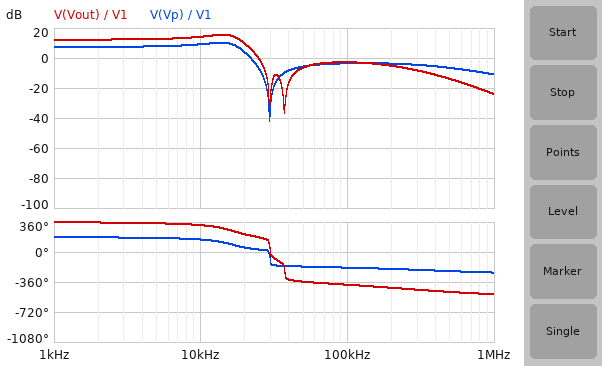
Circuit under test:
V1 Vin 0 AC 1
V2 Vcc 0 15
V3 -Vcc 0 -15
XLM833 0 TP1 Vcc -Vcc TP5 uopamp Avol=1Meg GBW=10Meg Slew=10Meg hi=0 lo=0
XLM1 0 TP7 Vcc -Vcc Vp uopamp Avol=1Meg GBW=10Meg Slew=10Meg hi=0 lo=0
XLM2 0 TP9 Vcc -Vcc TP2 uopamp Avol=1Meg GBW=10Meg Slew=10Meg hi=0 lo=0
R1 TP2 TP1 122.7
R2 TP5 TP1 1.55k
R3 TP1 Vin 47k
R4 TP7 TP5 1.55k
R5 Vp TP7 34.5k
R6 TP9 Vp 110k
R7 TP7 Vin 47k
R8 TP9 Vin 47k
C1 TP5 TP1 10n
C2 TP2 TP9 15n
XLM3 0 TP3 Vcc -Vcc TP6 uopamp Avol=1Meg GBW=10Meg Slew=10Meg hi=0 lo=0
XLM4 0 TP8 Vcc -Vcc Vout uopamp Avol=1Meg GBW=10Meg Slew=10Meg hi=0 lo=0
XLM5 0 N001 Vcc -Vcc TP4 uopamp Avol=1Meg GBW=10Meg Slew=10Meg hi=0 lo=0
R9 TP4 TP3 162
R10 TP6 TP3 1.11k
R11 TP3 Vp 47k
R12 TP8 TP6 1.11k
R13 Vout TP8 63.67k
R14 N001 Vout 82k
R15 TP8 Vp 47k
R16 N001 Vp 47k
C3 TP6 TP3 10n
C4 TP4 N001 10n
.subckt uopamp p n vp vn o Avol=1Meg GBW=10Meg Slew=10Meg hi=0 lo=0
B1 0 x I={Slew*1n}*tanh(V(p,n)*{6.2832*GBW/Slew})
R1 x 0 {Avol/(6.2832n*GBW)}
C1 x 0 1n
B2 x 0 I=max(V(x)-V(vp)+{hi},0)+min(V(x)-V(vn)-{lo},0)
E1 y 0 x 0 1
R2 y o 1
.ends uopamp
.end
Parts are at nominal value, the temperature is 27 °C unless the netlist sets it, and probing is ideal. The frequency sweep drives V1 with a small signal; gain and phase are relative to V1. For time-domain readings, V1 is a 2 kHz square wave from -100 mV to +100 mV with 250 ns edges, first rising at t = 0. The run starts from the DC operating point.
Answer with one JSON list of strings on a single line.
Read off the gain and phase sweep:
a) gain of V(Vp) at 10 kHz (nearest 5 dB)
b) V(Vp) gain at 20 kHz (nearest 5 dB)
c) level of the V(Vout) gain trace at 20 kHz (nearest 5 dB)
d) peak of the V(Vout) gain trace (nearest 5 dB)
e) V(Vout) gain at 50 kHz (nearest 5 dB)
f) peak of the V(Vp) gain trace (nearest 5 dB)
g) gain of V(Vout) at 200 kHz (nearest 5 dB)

["10 dB", "5 dB", "10 dB", "15 dB", "-5 dB", "10 dB", "-5 dB"]
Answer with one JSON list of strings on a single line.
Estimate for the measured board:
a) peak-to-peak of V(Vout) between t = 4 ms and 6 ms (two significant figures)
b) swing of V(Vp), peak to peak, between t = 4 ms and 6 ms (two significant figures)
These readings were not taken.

["1.3 V", "730 mV"]
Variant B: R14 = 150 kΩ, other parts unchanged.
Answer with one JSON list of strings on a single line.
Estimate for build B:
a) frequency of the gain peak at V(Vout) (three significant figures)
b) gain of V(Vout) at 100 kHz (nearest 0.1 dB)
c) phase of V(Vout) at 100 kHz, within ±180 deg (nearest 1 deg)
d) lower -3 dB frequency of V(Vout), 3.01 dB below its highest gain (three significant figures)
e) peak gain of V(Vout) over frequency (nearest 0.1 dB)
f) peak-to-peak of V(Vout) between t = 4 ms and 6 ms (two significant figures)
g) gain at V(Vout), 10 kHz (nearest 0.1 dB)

["14.9 kHz", "-3.2 dB", "-32 deg", "8.03 kHz", "22.1 dB", "2.7 V", "20.0 dB"]
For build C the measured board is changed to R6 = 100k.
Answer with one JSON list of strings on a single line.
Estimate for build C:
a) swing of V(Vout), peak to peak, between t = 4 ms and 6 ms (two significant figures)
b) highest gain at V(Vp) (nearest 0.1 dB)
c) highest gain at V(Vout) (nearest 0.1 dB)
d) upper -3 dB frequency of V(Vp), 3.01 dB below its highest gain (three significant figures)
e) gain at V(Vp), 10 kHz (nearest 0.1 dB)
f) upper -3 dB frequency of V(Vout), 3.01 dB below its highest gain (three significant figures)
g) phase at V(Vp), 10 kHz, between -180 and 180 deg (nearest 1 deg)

["1.2 V", "9.5 dB", "14.8 dB", "18.7 kHz", "8.2 dB", "19.0 kHz", "154 deg"]
